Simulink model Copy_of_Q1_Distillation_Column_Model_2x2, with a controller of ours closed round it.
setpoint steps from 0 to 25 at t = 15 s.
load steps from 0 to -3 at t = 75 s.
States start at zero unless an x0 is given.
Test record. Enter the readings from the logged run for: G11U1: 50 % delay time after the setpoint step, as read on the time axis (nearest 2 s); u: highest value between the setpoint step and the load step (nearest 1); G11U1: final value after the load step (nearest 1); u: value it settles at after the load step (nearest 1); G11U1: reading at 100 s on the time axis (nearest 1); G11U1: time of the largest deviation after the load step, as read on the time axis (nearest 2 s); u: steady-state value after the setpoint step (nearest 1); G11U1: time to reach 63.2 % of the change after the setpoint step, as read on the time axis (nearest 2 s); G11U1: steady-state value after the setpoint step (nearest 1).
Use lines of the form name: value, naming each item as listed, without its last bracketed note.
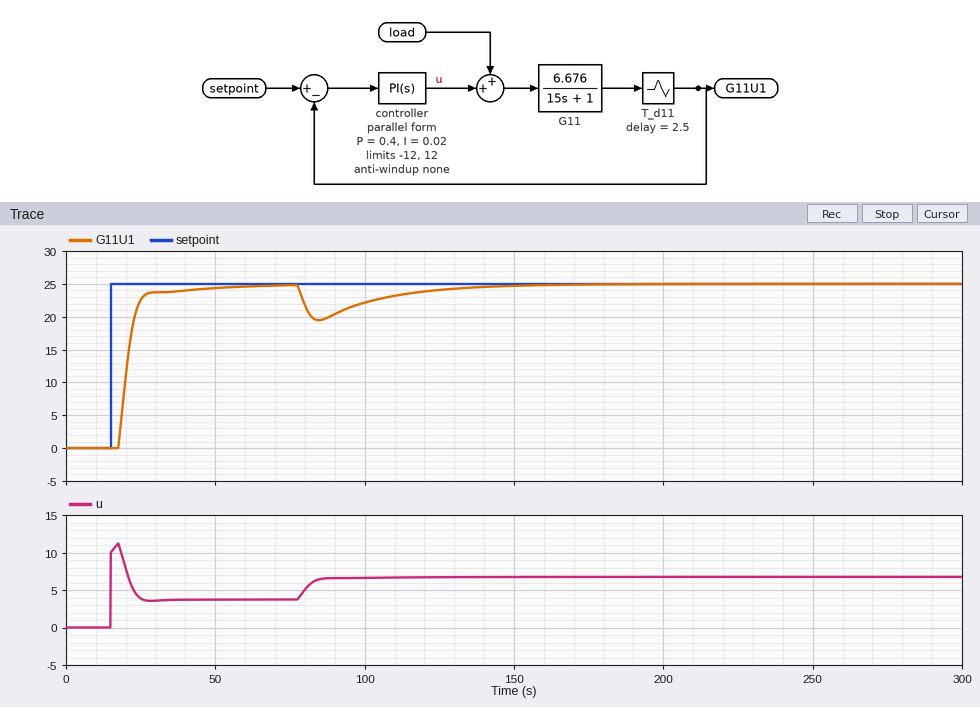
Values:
G11U1: 50 % delay time after the setpoint step, as read on the time axis: 20 s
u: highest value between the setpoint step and the load step: 11
G11U1: final value after the load step: 25
u: value it settles at after the load step: 7
G11U1: reading at 100 s on the time axis: 22
G11U1: time of the largest deviation after the load step, as read on the time axis: 84 s
u: steady-state value after the setpoint step: 4
G11U1: time to reach 63.2 % of the change after the setpoint step, as read on the time axis: 22 s
G11U1: steady-state value after the setpoint step: 25
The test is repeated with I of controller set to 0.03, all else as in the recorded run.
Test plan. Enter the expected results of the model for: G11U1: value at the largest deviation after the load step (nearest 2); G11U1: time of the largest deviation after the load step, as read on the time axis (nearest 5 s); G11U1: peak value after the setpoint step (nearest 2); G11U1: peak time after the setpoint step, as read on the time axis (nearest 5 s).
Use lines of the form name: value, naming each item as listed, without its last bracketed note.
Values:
G11U1: value at the largest deviation after the load step: 20
G11U1: time of the largest deviation after the load step, as read on the time axis: 85 s
G11U1: peak value after the setpoint step: 26
G11U1: peak time after the setpoint step, as read on the time axis: 30 s
